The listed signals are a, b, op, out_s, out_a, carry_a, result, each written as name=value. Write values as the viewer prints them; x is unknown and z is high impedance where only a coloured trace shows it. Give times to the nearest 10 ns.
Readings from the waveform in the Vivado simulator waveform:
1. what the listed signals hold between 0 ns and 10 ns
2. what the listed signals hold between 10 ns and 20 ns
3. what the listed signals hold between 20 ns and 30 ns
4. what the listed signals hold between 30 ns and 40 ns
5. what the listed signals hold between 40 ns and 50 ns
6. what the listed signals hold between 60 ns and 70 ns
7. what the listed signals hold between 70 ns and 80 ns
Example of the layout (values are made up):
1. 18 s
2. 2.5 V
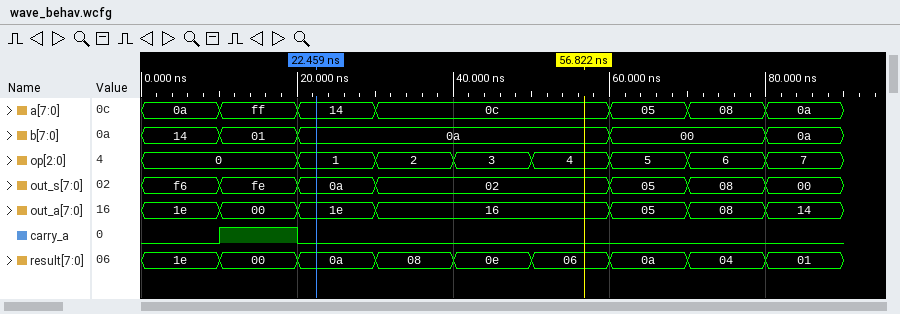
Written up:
1. a=0a, b=14, op=0, out_s=f6, out_a=1e, carry_a=0, result=1e
2. a=ff, b=01, op=0, out_s=fe, out_a=00, carry_a=1, result=00
3. a=14, b=0a, op=1, out_s=0a, out_a=1e, carry_a=0, result=0a
4. a=0c, b=0a, op=2, out_s=02, out_a=16, carry_a=0, result=08
5. a=0c, b=0a, op=3, out_s=02, out_a=16, carry_a=0, result=0e
6. a=05, b=00, op=5, out_s=05, out_a=05, carry_a=0, result=0a
7. a=08, b=00, op=6, out_s=08, out_a=08, carry_a=0, result=04
